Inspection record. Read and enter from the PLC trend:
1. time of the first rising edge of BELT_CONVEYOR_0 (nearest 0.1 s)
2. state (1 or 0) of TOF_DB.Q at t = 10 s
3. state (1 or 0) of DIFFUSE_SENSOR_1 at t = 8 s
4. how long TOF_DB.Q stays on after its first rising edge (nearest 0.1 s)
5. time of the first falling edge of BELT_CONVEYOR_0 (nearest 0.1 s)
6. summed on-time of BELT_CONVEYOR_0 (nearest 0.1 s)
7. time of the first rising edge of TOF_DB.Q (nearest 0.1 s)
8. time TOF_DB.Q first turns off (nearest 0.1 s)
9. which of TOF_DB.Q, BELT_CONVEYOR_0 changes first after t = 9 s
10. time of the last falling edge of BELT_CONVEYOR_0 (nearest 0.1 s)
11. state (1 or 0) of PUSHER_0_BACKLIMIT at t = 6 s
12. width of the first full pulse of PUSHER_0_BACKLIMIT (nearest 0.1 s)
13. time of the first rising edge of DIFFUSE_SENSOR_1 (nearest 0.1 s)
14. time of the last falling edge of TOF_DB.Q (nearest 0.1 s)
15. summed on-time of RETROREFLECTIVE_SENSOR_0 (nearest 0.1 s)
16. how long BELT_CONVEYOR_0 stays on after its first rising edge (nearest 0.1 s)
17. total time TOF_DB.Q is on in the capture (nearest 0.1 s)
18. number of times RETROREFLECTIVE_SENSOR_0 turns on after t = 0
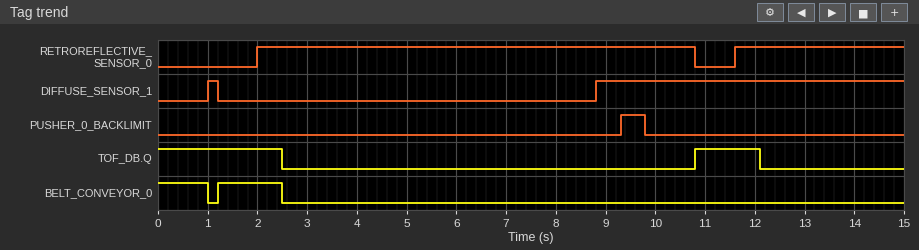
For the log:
1.2 s
0
0
1.3 s
1.0 s
2.3 s
10.8 s
2.5 s
TOF_DB.Q
2.5 s
0
0.5 s
1.0 s
12.1 s
12.2 s
1.3 s
3.8 s
2
